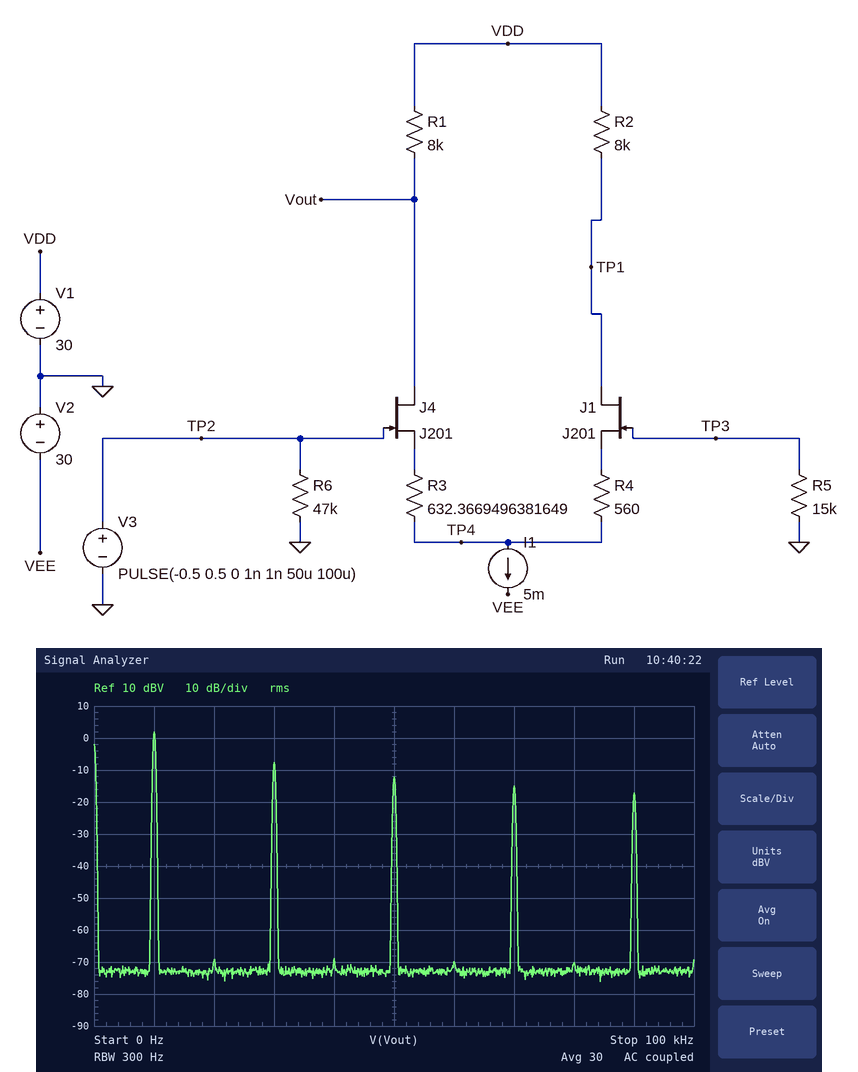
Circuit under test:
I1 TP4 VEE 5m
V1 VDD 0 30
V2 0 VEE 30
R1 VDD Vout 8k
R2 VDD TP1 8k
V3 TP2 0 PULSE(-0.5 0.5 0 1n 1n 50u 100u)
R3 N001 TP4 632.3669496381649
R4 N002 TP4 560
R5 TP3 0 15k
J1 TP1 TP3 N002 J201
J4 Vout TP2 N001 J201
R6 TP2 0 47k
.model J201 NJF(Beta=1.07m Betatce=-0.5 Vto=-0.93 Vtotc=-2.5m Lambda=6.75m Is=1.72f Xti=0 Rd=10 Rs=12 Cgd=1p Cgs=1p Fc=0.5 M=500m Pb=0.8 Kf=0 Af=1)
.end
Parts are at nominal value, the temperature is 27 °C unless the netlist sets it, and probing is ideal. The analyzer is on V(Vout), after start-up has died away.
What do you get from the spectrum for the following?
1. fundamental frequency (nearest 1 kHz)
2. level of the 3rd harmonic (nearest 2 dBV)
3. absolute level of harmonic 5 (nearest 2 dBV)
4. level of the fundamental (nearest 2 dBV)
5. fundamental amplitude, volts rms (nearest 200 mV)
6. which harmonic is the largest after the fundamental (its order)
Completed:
10 kHz
-8 dBV
-12 dBV
2 dBV
1.2 V
3
